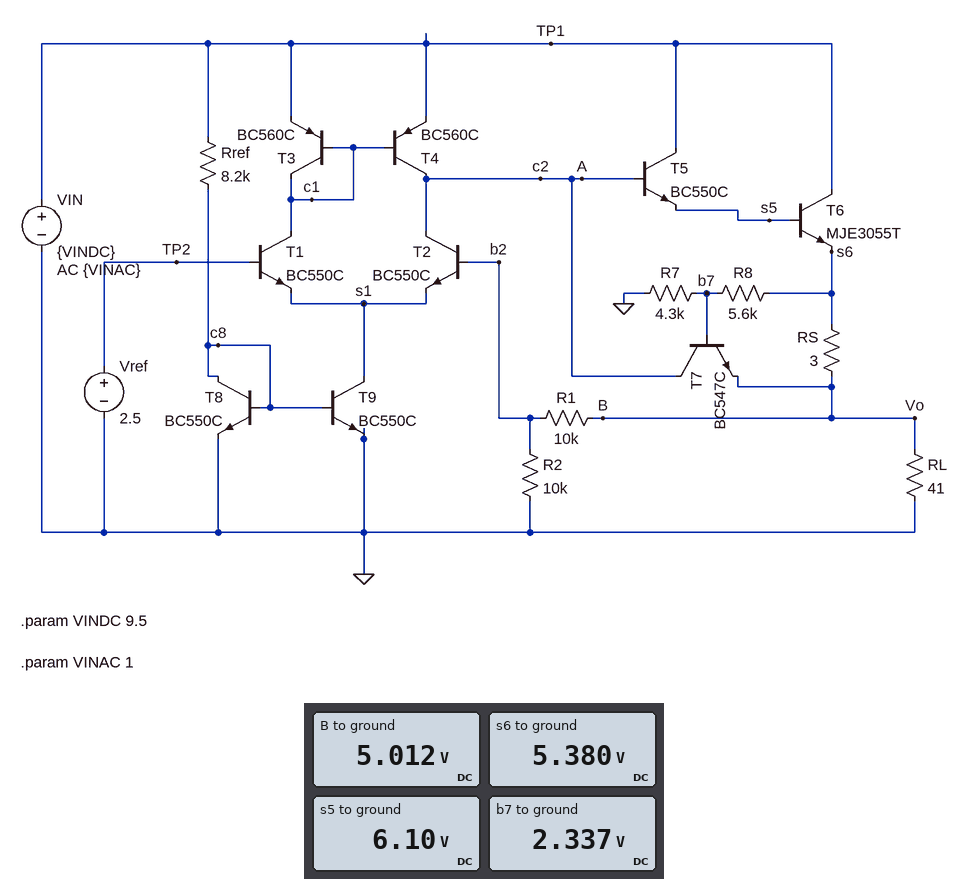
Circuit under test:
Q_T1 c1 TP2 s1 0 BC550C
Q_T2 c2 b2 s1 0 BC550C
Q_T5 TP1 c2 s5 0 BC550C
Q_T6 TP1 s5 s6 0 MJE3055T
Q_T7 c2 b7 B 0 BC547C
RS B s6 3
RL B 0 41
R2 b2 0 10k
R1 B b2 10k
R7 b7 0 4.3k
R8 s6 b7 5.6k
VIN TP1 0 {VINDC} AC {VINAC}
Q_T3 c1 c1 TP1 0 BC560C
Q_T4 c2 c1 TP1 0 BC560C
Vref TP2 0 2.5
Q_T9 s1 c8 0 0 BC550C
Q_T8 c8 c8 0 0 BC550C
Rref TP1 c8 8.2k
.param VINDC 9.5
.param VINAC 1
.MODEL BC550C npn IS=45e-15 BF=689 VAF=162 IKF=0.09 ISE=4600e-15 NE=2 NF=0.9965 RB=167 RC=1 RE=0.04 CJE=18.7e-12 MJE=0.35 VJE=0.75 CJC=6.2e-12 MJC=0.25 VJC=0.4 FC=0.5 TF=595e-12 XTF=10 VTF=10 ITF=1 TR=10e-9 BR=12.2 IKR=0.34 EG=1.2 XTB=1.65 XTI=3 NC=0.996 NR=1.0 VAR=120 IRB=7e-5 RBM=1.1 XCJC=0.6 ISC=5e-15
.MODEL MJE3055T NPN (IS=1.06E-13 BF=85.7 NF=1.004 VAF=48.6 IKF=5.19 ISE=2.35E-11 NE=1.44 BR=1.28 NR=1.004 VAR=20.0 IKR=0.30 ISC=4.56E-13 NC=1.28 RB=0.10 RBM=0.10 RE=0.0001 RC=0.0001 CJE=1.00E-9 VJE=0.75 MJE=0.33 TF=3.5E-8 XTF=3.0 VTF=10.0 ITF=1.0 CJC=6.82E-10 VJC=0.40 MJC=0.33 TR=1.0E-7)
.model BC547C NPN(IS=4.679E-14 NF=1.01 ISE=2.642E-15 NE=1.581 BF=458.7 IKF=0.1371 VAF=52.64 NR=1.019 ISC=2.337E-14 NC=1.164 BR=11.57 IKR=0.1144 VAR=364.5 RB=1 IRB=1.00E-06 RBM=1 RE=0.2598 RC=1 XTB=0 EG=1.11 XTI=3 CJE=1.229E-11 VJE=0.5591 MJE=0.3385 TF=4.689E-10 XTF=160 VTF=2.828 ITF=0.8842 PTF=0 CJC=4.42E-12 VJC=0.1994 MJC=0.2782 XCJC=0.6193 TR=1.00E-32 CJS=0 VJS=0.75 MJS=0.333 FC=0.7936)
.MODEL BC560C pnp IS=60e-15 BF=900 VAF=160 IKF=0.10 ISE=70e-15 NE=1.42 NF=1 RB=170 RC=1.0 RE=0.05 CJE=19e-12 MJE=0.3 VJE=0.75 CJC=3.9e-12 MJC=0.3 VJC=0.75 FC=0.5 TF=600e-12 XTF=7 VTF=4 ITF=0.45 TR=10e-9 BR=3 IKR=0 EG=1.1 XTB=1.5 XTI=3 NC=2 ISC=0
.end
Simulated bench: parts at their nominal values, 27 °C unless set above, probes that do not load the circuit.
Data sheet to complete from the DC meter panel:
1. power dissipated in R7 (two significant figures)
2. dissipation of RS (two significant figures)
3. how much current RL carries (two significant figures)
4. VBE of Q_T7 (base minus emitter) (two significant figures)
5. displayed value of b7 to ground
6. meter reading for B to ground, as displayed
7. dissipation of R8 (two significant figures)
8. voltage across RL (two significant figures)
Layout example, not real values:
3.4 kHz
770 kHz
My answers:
1.3 mW
45 mW
120 mA
-2.7 V
2.337 V
5.012 V
1.7 mW
5.0 V
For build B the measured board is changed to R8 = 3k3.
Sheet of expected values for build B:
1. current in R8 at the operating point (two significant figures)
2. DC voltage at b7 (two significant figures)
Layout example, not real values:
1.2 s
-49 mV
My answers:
710 µA
3.0 V
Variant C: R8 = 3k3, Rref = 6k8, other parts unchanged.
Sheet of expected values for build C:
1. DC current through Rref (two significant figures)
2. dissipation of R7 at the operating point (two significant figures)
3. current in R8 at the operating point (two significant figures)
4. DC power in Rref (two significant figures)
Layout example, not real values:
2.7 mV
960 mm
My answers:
1.3 mA
2.2 mW
710 µA
12 mW
